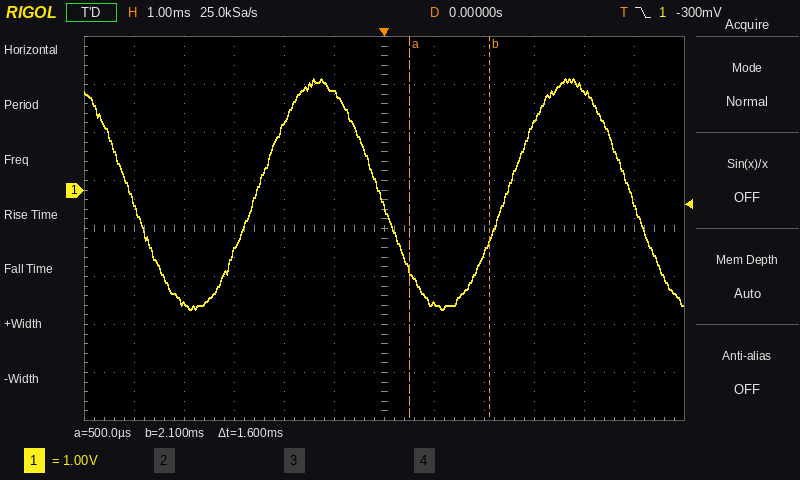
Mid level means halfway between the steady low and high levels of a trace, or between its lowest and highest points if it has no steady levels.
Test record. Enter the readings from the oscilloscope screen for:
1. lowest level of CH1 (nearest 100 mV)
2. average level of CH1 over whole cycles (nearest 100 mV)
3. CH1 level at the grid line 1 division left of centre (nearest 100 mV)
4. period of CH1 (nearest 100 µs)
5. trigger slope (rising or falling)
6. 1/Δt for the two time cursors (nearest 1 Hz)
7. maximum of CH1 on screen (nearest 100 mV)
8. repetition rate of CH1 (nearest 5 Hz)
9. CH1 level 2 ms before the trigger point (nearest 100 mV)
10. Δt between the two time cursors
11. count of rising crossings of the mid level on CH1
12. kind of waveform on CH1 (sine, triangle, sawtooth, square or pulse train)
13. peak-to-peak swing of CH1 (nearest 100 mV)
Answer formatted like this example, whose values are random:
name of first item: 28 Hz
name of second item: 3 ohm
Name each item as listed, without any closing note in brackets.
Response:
lowest level of CH1: -2.5 V
average level of CH1 over whole cycles: -100 mV
CH1 level at the grid line 1 division left of centre: 2.0 V
period of CH1: 5.0 ms
trigger slope: falling
1/Δt for the two time cursors: 625 Hz
maximum of CH1 on screen: 2.3 V
repetition rate of CH1: 200 Hz
CH1 level 2 ms before the trigger point: 1.4 V
Δt between the two time cursors: 1.6 ms
count of rising crossings of the mid level on CH1: 2
kind of waveform on CH1: sine
peak-to-peak swing of CH1: 4.8 V
